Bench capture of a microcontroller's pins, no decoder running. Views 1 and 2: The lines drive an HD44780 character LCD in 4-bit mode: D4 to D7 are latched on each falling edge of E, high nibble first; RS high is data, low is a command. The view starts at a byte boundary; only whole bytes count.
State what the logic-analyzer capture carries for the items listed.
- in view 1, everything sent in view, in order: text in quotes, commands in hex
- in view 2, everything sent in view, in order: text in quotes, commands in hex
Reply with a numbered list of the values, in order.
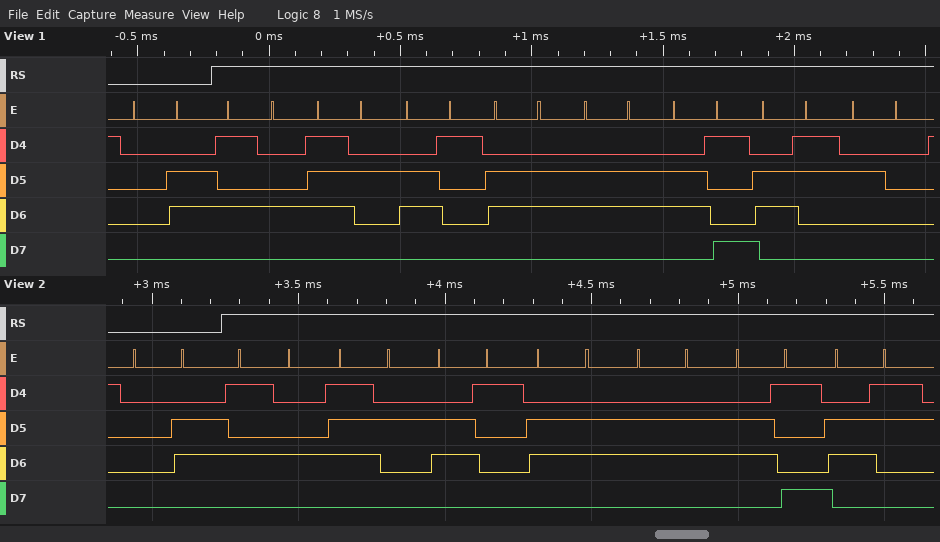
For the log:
1. 0x06 "Traffic "
2. 0x06 "Traffic"
